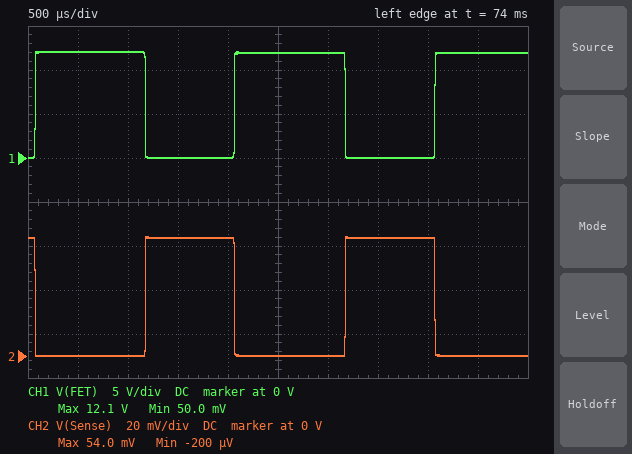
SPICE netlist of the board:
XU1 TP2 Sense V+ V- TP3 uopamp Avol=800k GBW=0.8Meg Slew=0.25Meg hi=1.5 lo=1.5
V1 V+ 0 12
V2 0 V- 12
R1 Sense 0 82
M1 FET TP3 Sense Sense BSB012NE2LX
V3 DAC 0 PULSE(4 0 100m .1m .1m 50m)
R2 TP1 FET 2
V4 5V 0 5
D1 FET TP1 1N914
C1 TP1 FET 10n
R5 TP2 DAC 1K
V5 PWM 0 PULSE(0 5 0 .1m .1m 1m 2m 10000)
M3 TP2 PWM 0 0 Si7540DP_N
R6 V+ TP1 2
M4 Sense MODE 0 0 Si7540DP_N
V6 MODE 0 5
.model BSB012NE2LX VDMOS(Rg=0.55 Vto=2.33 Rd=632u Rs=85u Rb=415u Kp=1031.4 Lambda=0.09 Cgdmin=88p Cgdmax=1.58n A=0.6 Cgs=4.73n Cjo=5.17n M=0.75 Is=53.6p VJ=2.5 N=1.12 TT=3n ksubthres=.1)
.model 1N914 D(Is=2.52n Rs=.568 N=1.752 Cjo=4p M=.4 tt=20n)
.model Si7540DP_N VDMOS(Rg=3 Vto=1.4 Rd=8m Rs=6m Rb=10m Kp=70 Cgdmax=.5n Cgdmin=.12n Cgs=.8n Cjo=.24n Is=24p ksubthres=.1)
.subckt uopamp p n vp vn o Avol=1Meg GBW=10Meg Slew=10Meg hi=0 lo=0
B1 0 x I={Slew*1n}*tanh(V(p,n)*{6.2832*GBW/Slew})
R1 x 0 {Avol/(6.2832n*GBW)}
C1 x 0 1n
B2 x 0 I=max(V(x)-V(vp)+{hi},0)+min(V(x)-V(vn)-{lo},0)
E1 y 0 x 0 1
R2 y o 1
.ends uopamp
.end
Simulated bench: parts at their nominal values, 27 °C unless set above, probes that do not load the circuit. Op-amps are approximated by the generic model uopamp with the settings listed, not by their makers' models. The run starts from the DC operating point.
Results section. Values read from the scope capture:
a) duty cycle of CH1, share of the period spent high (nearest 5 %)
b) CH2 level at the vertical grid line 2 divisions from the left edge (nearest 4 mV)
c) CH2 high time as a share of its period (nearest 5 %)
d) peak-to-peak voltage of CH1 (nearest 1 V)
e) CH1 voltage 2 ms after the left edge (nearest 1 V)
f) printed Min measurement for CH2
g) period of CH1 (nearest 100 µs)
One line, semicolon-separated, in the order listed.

55 %; 0 V; 45 %; 12 V; 0 V; -200 µV; 2.0 ms
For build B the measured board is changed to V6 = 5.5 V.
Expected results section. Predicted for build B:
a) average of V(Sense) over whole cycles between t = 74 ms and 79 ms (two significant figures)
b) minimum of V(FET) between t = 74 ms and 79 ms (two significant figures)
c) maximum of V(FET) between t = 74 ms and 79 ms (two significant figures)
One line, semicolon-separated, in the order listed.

23 mV; 55 mV; 12 V
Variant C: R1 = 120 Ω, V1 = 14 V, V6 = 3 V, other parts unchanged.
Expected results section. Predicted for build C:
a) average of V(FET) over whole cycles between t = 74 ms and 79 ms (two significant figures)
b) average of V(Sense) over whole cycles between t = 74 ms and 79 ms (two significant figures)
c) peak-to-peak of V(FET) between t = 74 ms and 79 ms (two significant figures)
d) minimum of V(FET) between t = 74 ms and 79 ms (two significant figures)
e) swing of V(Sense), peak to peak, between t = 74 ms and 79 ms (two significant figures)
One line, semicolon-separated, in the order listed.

7.8 V; 36 mV; 14 V; 83 mV; 81 mV
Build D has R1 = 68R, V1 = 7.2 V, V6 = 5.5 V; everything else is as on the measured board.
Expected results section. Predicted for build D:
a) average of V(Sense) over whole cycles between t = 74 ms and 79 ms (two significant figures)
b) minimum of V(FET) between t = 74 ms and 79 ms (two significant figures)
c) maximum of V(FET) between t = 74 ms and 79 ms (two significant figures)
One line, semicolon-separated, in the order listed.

14 mV; 33 mV; 7.2 V
